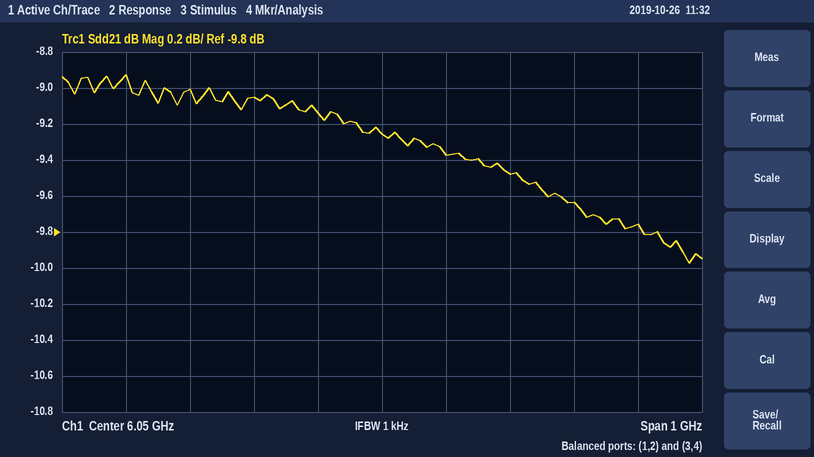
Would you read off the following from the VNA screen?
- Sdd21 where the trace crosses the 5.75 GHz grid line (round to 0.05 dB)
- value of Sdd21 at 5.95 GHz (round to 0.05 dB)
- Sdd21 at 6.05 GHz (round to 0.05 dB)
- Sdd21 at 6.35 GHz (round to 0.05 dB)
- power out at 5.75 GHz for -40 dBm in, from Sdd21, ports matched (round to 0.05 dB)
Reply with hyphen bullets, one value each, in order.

- -9.00 dB
- -9.15 dB
- -9.25 dB
- -9.65 dB
- -49.00 dBm
